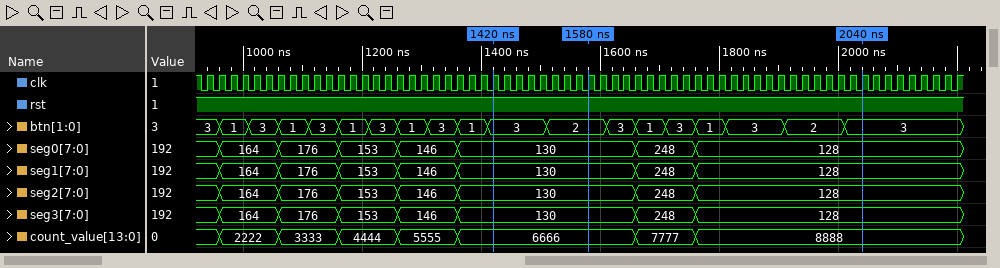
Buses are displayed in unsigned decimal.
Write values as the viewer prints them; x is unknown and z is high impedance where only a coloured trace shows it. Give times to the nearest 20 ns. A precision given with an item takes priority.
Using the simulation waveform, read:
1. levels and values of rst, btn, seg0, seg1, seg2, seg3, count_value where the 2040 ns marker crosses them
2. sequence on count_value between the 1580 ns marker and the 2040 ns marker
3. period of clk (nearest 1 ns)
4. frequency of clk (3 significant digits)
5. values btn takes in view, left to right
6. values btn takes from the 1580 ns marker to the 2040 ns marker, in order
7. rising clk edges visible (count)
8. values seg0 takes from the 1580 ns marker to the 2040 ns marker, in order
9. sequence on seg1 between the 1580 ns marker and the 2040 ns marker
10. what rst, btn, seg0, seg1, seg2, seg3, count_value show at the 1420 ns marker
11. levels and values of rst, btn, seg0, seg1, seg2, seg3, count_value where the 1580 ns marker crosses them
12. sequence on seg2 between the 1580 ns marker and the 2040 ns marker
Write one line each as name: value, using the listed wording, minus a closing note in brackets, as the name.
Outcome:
levels and values of rst, btn, seg0, seg1, seg2, seg3, count_value where the 2040 ns marker crosses them: rst=1, btn=3, seg0=128, seg1=128, seg2=128, seg3=128, count_value=8888
sequence on count_value between the 1580 ns marker and the 2040 ns marker: 6666, 7777, 8888
period of clk: 20 ns
frequency of clk: 50.0 MHz
values btn takes in view, left to right: 3, 1, 3, 1, 3, 1, 3, 1, 3, 1, 3, 2, 3, 1, 3, 1, 3, 2, 3
values btn takes from the 1580 ns marker to the 2040 ns marker, in order: 2, 3, 1, 3, 1, 3, 2, 3
rising clk edges visible: 64
values seg0 takes from the 1580 ns marker to the 2040 ns marker, in order: 130, 248, 128
sequence on seg1 between the 1580 ns marker and the 2040 ns marker: 130, 248, 128
what rst, btn, seg0, seg1, seg2, seg3, count_value show at the 1420 ns marker: rst=1, btn=3, seg0=130, seg1=130, seg2=130, seg3=130, count_value=6666
levels and values of rst, btn, seg0, seg1, seg2, seg3, count_value where the 1580 ns marker crosses them: rst=1, btn=2, seg0=130, seg1=130, seg2=130, seg3=130, count_value=6666
sequence on seg2 between the 1580 ns marker and the 2040 ns marker: 130, 248, 128
